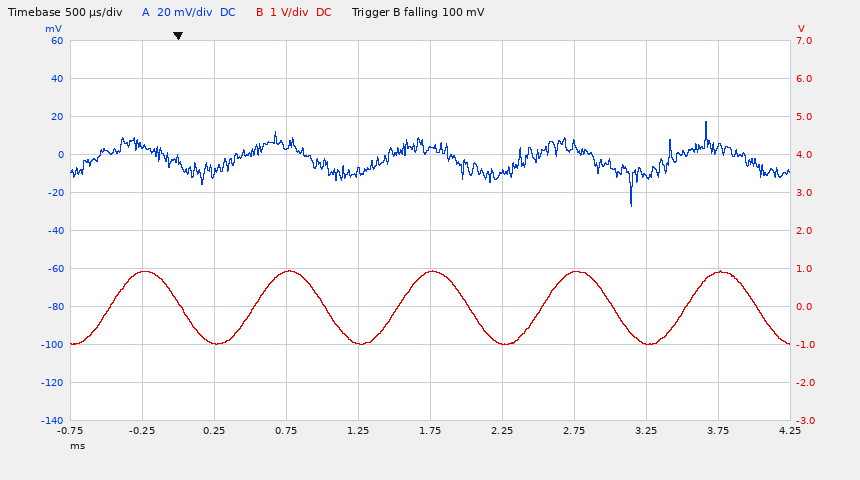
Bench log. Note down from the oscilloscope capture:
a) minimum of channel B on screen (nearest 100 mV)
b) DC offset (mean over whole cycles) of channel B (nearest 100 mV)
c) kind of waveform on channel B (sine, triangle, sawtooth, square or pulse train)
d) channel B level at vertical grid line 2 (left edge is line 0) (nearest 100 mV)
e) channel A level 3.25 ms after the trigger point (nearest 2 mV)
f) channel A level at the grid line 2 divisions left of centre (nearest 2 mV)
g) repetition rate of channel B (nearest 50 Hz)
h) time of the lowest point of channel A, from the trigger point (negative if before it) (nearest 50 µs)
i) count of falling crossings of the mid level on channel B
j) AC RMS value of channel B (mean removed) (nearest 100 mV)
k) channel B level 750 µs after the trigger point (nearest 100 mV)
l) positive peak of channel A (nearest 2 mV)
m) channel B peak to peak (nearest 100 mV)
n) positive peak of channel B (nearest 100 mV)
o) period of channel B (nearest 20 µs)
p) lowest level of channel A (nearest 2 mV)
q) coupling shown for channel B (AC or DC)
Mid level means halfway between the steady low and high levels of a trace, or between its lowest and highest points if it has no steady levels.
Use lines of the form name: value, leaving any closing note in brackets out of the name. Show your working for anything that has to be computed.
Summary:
minimum of channel B on screen: -1.0 V
DC offset (mean over whole cycles) of channel B: (900 mV + (-1.0 V)) / 2 ≈ 0.0 V
kind of waveform on channel B: sine
channel B level at vertical grid line 2 (left edge is line 0): -1.0 V
channel A level 3.25 ms after the trigger point: -12 mV
channel A level at the grid line 2 divisions left of centre: 4 mV
repetition rate of channel B: 1 / 1.00 ms ≈ 1.00 kHz
time of the lowest point of channel A, from the trigger point (negative if before it): +3.15 ms
count of falling crossings of the mid level on channel B: 5
AC RMS value of channel B (mean removed): 1.9 V / (2√2) ≈ 672 mV, so 700 mV to the nearest 100 mV
channel B level 750 µs after the trigger point: 900 mV
positive peak of channel A: 18 mV
channel B peak to peak: 900 mV − (-1.0 V) = 1.9 V
positive peak of channel B: 900 mV
period of channel B: 1.00 ms
lowest level of channel A: -28 mV
coupling shown for channel B: DC
